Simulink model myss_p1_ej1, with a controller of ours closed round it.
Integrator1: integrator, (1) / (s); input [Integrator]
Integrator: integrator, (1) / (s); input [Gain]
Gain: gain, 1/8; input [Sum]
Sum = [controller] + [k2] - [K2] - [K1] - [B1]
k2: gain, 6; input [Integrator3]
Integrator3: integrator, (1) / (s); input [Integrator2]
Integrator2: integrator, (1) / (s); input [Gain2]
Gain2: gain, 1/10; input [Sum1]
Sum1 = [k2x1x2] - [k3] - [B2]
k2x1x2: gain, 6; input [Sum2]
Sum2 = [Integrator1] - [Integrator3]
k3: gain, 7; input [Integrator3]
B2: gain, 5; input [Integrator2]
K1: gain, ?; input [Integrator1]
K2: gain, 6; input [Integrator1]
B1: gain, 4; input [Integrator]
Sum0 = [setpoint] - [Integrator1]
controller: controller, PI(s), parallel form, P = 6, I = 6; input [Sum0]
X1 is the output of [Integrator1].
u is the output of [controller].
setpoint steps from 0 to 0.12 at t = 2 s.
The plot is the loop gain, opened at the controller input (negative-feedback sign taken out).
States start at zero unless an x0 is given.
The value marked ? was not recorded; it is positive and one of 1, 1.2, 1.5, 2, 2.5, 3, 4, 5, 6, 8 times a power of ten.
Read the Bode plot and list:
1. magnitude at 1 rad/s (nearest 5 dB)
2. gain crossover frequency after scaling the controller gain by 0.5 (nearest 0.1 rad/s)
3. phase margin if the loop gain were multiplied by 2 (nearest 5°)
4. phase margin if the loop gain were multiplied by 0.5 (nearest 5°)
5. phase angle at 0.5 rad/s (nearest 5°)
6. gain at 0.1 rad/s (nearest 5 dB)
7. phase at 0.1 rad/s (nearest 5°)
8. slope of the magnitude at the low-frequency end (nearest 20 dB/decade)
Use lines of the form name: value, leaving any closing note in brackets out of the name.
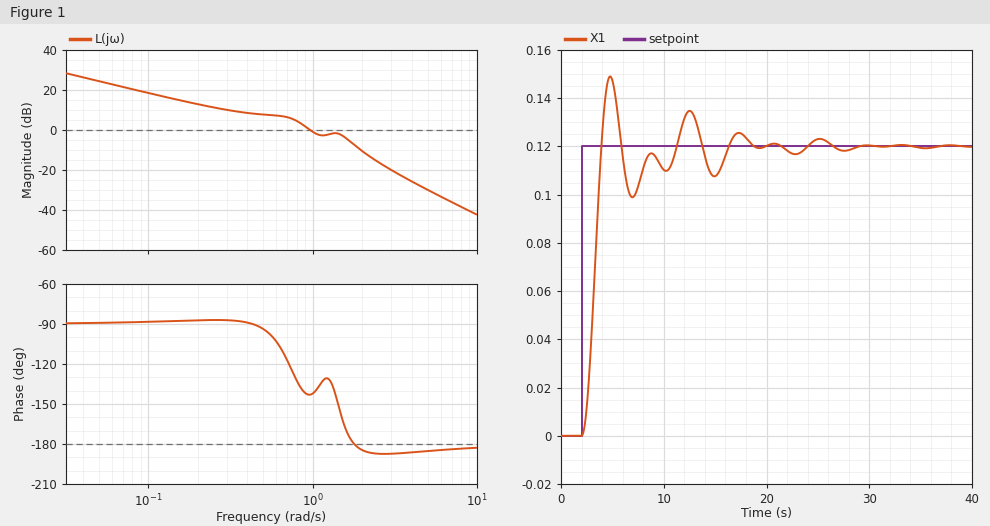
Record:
magnitude at 1 rad/s: 0 dB
gain crossover frequency after scaling the controller gain by 0.5: 0.7 rad/s
phase margin if the loop gain were multiplied by 2: 5°
phase margin if the loop gain were multiplied by 0.5: 60°
phase angle at 0.5 rad/s: -95°
gain at 0.1 rad/s: 20 dB
phase at 0.1 rad/s: -90°
slope of the magnitude at the low-frequency end: -20 dB/decade
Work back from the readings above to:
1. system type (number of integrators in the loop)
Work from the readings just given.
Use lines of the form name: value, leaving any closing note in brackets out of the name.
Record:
system type: 1
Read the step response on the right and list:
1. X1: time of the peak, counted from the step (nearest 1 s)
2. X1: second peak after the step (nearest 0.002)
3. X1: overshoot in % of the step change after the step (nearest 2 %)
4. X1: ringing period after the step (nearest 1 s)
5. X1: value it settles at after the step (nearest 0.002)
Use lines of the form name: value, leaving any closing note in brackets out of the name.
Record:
X1: time of the peak, counted from the step: 3 s
X1: second peak after the step: 0.134
X1: overshoot in % of the step change after the step: 24 %
X1: ringing period after the step: 8 s
X1: value it settles at after the step: 0.120
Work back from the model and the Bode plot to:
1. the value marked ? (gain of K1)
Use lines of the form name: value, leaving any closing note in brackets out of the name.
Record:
the value marked ?: 4
